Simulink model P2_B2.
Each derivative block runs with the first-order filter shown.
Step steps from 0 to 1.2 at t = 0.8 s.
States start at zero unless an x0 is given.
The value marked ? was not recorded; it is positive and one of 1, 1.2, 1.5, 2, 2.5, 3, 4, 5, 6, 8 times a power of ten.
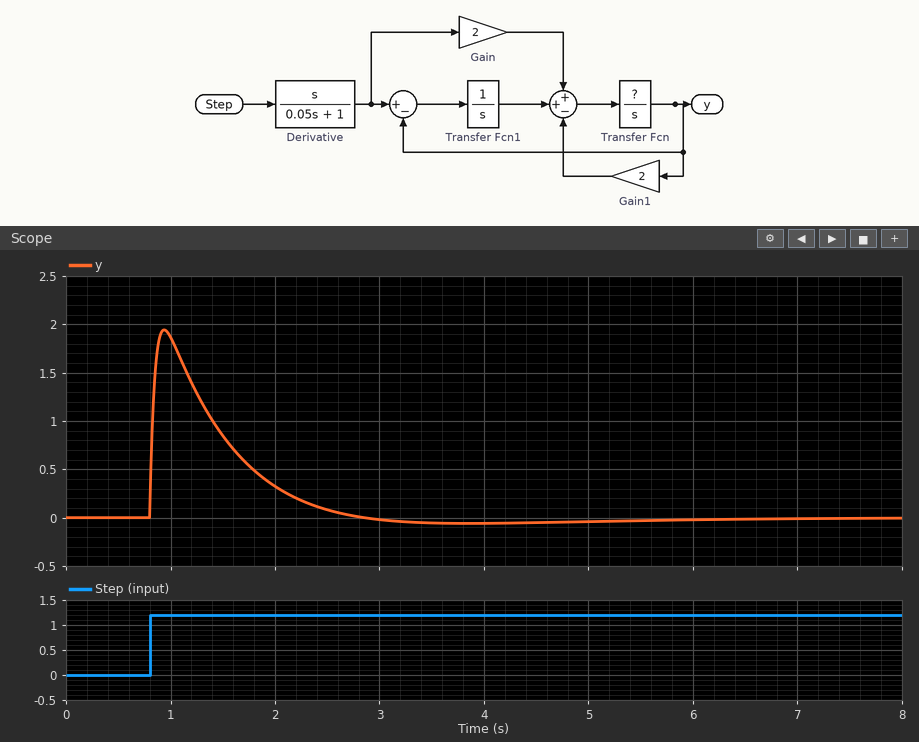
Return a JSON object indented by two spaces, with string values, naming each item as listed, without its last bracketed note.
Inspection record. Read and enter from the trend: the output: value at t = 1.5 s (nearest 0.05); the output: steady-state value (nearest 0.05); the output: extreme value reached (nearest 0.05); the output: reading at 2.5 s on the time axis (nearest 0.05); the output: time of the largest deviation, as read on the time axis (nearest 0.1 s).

{
  "the output: value at t = 1.5 s": "0.85",
  "the output: steady-state value": "0.00",
  "the output: extreme value reached": "1.95",
  "the output: reading at 2.5 s on the time axis": "0.10",
  "the output: time of the largest deviation, as read on the time axis": "0.9 s"
}
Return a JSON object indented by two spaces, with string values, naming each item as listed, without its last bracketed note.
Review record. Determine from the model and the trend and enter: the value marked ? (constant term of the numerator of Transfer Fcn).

{
  "the value marked ?": "1"
}
